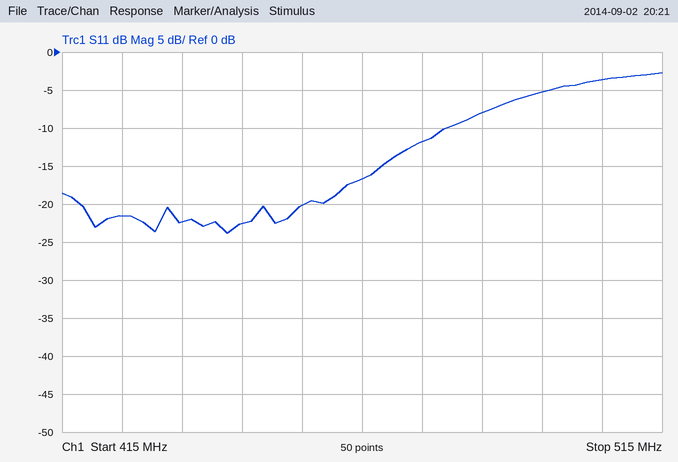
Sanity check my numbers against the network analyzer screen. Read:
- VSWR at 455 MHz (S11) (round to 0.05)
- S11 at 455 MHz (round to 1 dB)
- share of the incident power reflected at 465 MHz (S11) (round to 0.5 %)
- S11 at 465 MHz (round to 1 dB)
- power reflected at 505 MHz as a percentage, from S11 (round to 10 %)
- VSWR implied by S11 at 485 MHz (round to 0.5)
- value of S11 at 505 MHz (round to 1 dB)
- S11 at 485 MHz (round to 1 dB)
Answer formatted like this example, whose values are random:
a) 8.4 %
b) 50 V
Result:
a) 1.20
b) -20 dB
c) 2.0 %
d) -17 dB
e) 40 %
f) 2.5
g) -4 dB
h) -8 dB
